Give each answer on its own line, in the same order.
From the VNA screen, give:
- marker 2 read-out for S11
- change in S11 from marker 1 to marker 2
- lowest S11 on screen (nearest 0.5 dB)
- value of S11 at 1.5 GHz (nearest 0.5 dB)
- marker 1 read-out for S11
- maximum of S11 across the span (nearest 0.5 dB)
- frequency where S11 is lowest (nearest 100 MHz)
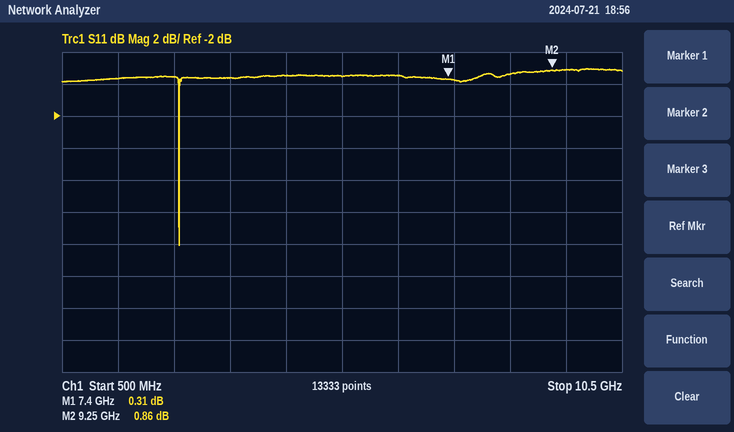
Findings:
0.86 dB
0.55 dB
-10.0 dB
0.5 dB
0.31 dB
1.0 dB
2.6 GHz
